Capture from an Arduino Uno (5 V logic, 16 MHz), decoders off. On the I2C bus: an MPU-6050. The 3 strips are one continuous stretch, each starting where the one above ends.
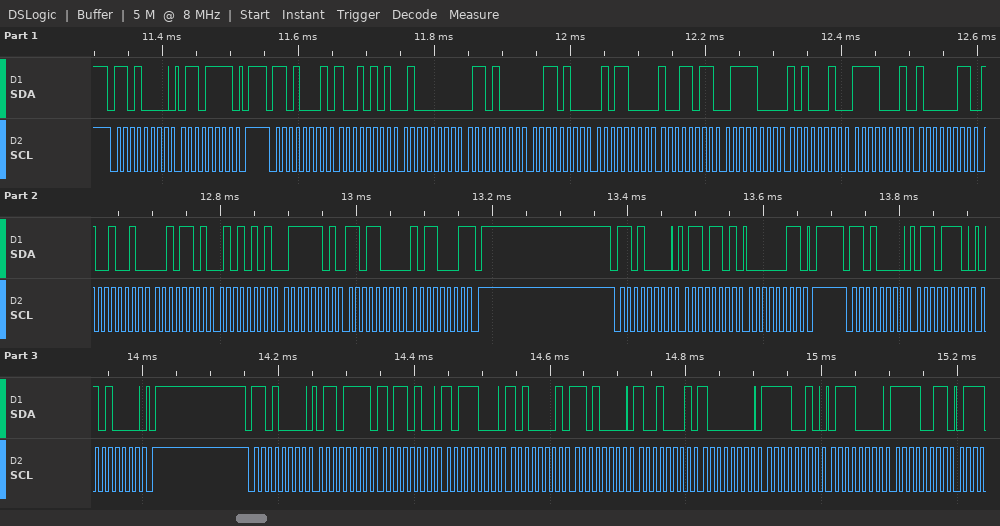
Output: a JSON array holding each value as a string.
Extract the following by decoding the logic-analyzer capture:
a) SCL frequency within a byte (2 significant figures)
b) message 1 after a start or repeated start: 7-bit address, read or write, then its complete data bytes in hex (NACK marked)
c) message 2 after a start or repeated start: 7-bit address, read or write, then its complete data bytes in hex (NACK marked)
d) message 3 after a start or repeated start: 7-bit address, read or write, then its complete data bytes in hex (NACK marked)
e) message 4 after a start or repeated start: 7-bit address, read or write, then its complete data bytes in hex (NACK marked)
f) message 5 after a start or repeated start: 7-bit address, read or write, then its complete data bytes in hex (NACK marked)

["100 kHz", "0x68 write: 6F", "0x68 read: 95 40 68 34 58 9B 78 A2 F1 83 92 2D 55 7D D8 B1 NACK", "0x68 write: 6D 03", "0x68 write: 6E 50", "0x68 write: 6F B4 B8 A1 D0 91 80 F2 70 F3"]
